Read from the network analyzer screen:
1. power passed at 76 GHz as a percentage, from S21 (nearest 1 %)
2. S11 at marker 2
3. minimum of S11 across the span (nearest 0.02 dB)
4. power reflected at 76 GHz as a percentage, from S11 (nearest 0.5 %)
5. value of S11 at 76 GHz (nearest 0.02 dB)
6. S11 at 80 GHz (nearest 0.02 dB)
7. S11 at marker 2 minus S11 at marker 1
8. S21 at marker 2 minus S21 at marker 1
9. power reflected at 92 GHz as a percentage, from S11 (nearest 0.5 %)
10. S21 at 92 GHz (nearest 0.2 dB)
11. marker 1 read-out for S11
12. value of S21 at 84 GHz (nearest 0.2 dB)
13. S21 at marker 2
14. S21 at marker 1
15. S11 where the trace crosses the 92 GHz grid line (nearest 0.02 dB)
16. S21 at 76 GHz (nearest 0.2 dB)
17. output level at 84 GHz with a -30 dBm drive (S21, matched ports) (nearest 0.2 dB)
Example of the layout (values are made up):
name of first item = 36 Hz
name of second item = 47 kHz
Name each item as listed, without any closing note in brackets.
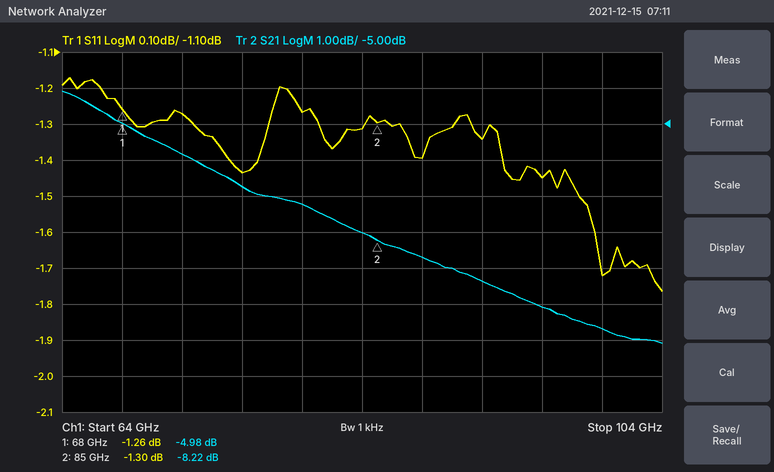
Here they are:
power passed at 76 GHz as a percentage, from S21 = 21 %
S11 at marker 2 = -1.30 dB
minimum of S11 across the span = -1.76 dB
power reflected at 76 GHz as a percentage, from S11 = 72.0 %
value of S11 at 76 GHz = -1.44 dB
S11 at 80 GHz = -1.26 dB
S11 at marker 2 minus S11 at marker 1 = -0.04 dB
S21 at marker 2 minus S21 at marker 1 = -3.24 dB
power reflected at 92 GHz as a percentage, from S11 = 73.5 %
S21 at 92 GHz = -9.4 dB
marker 1 read-out for S11 = -1.26 dB
value of S21 at 84 GHz = -8.0 dB
S21 at marker 2 = -8.22 dB
S21 at marker 1 = -4.98 dB
S11 where the trace crosses the 92 GHz grid line = -1.34 dB
S21 at 76 GHz = -6.8 dB
output level at 84 GHz with a -30 dBm drive (S21, matched ports) = -38.0 dBm
